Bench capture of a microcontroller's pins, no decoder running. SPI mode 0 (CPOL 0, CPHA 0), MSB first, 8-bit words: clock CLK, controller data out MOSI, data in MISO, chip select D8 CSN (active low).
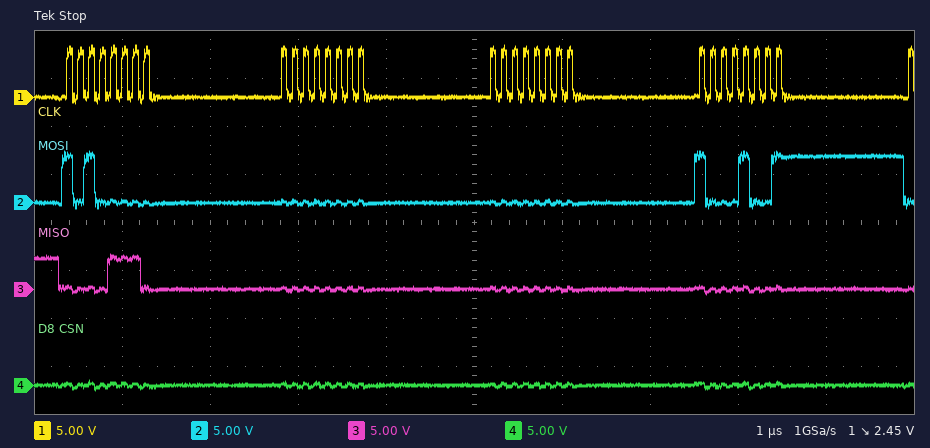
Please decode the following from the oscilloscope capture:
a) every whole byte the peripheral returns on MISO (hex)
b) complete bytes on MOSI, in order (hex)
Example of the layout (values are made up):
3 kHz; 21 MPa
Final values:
0x0E 0x00 0x00 0x00; 0xA0 0x00 0x00 0x89
